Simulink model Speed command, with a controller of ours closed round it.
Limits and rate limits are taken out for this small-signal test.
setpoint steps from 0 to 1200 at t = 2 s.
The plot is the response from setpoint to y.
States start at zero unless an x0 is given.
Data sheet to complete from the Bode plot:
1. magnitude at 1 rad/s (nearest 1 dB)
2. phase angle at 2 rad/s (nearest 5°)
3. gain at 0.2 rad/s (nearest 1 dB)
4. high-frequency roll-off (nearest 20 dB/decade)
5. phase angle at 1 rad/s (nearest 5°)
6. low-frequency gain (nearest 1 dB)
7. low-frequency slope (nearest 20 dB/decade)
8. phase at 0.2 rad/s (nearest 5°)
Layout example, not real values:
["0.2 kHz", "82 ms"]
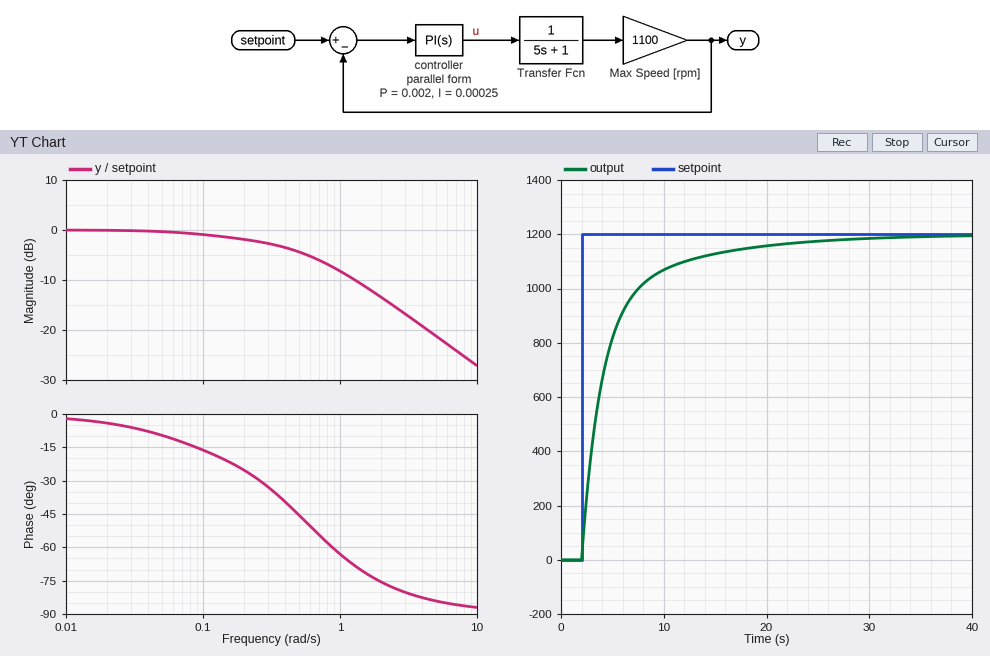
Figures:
["-8 dB", "-75°", "-2 dB", "-20 dB/decade", "-65°", "0 dB", "0 dB/decade", "-25°"]
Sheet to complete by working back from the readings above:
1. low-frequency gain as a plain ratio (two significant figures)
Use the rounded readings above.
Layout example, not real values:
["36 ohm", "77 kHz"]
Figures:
["1.0"]
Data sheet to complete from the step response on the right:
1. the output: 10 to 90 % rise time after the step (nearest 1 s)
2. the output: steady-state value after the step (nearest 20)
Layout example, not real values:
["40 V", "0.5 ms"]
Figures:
["8 s", "1200"]
